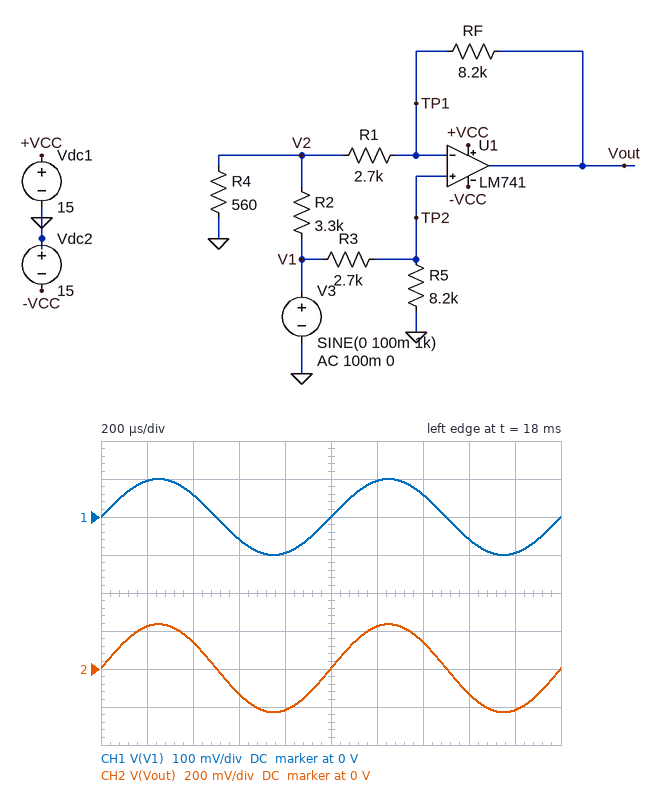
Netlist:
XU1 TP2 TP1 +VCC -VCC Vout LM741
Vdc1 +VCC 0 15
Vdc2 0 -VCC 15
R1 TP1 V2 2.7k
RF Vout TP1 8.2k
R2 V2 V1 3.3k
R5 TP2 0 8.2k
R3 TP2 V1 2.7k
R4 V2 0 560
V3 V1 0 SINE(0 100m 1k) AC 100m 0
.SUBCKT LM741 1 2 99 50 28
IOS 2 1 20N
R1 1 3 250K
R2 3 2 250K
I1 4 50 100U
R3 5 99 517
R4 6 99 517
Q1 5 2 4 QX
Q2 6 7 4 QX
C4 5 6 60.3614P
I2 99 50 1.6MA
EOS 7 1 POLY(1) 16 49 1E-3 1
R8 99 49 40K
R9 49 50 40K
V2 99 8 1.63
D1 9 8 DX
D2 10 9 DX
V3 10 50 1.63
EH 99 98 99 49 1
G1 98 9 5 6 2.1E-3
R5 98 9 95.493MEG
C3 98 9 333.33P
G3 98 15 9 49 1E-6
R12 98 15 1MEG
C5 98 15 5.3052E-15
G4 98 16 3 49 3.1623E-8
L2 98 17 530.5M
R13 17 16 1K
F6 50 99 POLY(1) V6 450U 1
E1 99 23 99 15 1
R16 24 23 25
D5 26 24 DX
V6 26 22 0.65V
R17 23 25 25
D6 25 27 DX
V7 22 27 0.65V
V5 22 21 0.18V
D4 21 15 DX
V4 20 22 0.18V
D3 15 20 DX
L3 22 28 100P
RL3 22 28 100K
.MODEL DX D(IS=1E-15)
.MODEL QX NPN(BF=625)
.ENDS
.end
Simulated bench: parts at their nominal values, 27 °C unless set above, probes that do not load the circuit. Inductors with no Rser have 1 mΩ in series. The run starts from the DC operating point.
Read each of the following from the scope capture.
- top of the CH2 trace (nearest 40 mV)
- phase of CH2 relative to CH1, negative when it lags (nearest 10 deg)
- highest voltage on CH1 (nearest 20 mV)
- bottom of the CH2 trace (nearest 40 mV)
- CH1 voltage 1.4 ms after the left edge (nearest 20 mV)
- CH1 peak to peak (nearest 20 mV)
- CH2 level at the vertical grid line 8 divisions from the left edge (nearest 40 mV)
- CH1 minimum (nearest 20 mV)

240 mV
0 deg
100 mV
-240 mV
60 mV
200 mV
-120 mV
-100 mV
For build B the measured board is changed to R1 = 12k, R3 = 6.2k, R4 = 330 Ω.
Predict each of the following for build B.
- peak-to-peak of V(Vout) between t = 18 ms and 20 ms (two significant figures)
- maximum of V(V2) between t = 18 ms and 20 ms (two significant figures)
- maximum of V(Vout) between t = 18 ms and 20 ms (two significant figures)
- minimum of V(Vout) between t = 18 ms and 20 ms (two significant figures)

180 mV
10 mV
91 mV
-87 mV
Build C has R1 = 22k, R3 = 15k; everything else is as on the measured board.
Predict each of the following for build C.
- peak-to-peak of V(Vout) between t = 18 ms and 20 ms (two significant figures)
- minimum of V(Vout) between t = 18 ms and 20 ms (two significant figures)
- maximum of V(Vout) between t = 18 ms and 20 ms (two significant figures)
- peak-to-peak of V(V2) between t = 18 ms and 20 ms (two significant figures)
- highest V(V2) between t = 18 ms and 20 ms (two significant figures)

86 mV
-41 mV
45 mV
30 mV
15 mV
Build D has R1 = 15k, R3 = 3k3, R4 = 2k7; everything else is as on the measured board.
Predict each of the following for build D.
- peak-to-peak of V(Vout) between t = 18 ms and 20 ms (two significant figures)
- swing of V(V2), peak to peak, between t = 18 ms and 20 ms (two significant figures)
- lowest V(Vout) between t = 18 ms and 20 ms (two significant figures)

170 mV
95 mV
-82 mV
